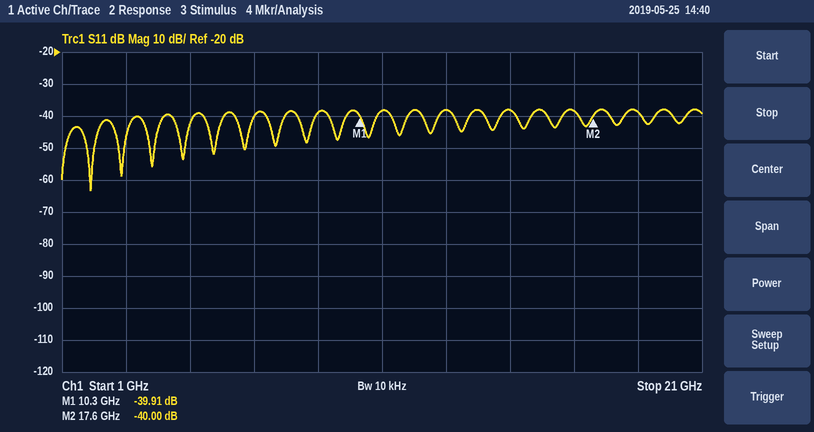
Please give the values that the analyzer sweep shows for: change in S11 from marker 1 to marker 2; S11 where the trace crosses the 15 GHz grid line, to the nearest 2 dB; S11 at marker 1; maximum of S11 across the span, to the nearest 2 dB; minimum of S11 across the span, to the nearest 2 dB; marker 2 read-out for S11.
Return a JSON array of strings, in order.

["-0.09 dB", "-38 dB", "-39.91 dB", "-38 dB", "-64 dB", "-40.00 dB"]
